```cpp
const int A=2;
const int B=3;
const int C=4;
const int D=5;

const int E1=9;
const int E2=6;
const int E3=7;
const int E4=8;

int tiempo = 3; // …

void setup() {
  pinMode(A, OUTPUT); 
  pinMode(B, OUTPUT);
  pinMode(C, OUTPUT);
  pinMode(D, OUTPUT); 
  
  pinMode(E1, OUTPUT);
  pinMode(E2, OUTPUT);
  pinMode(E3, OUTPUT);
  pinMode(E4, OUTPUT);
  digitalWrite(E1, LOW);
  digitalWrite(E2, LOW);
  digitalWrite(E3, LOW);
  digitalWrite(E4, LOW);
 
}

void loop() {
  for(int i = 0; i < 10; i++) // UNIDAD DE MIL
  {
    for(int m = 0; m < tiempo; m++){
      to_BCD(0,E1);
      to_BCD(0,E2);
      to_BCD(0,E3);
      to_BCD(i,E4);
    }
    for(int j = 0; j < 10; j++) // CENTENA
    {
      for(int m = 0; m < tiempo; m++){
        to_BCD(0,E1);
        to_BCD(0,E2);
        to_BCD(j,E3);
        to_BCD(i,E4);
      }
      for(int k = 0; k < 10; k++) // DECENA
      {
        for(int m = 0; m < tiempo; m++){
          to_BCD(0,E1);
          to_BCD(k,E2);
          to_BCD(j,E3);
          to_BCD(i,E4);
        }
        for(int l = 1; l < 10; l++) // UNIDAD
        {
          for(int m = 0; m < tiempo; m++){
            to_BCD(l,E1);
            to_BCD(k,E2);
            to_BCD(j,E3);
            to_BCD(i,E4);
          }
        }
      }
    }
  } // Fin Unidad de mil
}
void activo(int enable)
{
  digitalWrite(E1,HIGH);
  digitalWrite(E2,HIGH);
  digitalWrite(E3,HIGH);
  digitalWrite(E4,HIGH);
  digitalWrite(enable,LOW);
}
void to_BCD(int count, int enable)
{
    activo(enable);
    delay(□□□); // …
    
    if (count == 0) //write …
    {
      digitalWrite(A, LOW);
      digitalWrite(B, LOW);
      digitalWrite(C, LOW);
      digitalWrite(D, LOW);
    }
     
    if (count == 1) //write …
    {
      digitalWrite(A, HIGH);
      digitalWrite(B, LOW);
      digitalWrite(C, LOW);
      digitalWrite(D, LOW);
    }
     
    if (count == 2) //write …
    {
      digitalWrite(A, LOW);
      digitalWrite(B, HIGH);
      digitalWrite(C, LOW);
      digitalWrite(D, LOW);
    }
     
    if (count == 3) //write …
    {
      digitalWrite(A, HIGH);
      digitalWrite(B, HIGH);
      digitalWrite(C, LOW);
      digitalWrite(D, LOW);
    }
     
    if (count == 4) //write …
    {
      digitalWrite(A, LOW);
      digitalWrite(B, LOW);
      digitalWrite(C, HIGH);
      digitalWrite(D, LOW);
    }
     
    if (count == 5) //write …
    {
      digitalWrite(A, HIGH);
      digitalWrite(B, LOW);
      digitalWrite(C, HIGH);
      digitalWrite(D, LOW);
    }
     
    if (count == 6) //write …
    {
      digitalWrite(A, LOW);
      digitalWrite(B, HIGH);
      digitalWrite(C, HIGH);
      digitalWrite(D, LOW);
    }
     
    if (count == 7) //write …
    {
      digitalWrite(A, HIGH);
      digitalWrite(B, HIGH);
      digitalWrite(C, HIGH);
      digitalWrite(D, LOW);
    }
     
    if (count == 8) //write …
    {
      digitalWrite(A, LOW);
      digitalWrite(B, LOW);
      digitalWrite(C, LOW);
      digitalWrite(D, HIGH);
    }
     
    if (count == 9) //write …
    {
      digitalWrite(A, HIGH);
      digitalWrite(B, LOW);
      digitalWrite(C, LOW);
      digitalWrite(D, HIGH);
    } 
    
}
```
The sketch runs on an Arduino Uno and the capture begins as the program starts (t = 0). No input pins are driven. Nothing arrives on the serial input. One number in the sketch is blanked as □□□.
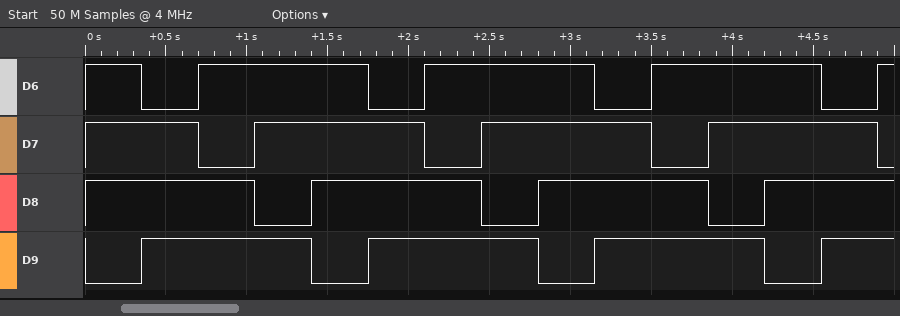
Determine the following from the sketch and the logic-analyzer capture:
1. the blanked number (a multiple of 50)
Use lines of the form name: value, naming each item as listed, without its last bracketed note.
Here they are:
the blanked number: 350
